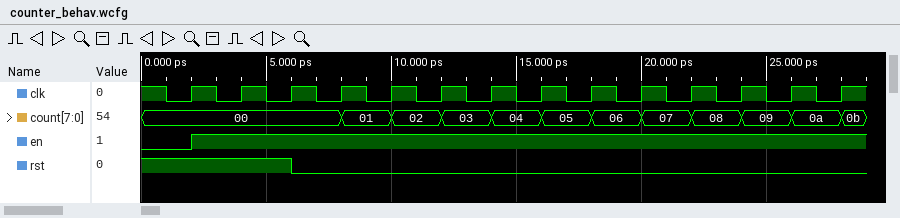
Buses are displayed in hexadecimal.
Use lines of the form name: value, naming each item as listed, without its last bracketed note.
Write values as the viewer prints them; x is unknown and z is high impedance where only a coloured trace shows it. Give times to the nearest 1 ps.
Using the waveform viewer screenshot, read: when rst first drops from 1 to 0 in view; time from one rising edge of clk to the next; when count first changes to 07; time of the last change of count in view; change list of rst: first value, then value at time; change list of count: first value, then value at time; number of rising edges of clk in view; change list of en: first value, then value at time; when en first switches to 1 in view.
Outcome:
when rst first drops from 1 to 0 in view: 6 ps
time from one rising edge of clk to the next: 2 ps
when count first changes to 07: 20 ps
time of the last change of count in view: 28 ps
change list of rst: first value, then value at time: 1, 0 at 6 ps
change list of count: first value, then value at time: 00, 01 at 8 ps, 02 at 10 ps, 03 at 12 ps, 04 at 14 ps, 05 at 16 ps, 06 at 18 ps, 07 at 20 ps, 08 at 22 ps, 09 at 24 ps, 0a at 26 ps, 0b at 28 ps
number of rising edges of clk in view: 14
change list of en: first value, then value at time: 0, 1 at 2 ps
when en first switches to 1 in view: 2 ps
